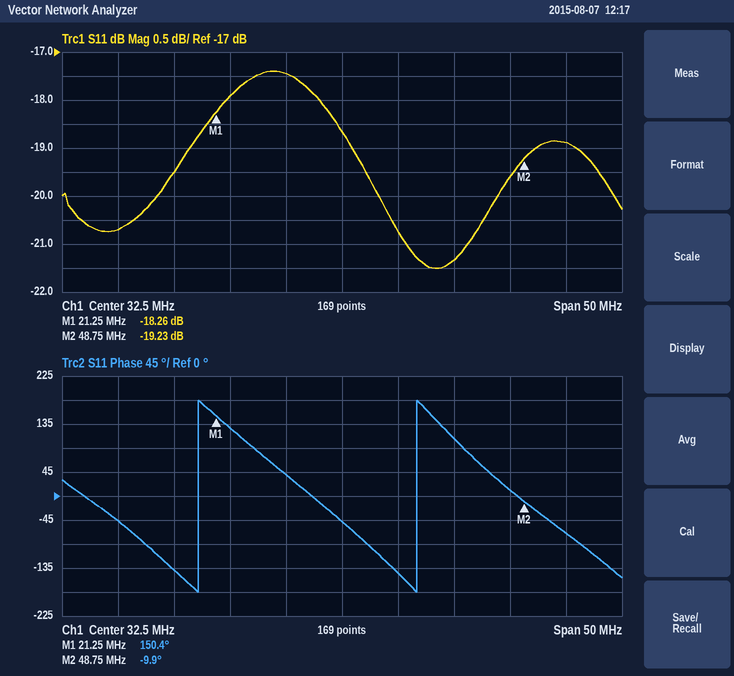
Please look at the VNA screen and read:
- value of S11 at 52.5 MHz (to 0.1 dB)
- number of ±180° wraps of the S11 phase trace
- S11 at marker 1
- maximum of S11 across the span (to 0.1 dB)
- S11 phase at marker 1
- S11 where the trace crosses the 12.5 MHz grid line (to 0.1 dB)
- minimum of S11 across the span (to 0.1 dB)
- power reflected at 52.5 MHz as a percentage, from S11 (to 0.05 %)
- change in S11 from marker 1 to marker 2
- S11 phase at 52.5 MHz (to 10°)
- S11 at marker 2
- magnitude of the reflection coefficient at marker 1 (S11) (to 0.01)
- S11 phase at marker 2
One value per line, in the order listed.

-18.9 dB
2
-18.26 dB
-17.4 dB
150.4°
-20.7 dB
-21.5 dB
1.30 %
-0.97 dB
-70°
-19.23 dB
0.12
-9.9°
